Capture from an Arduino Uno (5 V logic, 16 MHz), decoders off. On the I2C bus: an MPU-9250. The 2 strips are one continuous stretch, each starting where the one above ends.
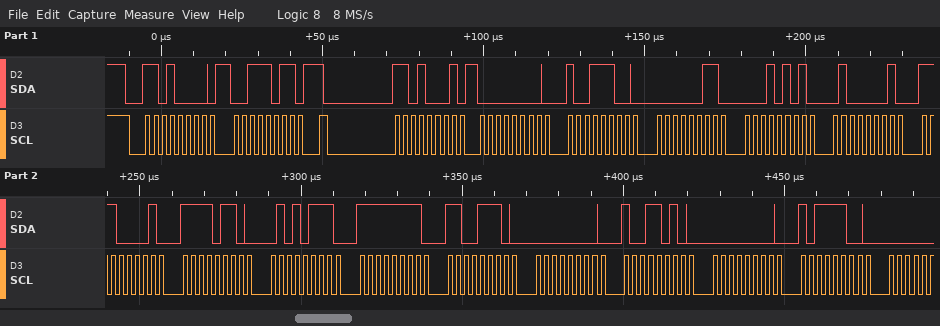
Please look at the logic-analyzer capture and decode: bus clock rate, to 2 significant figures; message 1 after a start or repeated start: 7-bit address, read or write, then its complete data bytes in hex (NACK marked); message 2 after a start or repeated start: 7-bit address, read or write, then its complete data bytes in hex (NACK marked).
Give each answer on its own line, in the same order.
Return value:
400 kHz
0x68 write: 3B
0x68 read: 00 9C 03 15 41 E1 F6 57 FF CE 00 9A 00 BC
